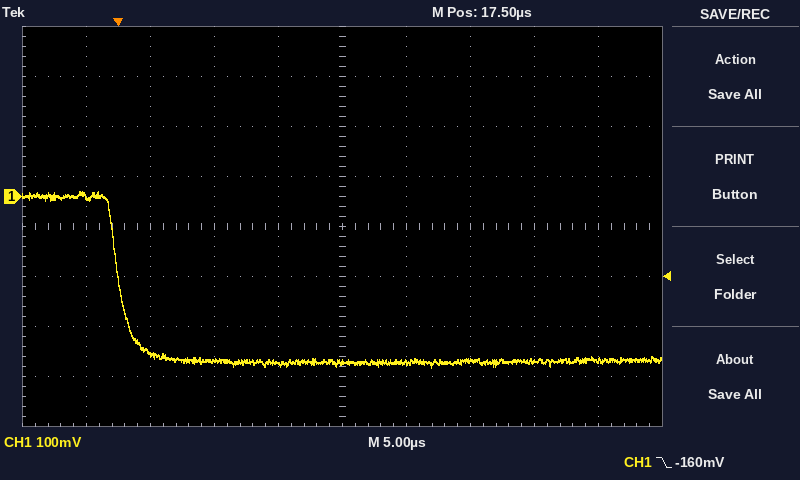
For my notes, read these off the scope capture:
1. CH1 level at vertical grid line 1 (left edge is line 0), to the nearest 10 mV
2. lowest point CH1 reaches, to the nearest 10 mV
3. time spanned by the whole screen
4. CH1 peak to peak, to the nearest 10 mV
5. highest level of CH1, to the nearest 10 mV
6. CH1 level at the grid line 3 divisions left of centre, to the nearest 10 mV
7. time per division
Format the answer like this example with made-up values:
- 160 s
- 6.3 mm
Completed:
- 0 mV
- -340 mV
- 50 µs
- 350 mV
- 10 mV
- -310 mV
- 5 µs
